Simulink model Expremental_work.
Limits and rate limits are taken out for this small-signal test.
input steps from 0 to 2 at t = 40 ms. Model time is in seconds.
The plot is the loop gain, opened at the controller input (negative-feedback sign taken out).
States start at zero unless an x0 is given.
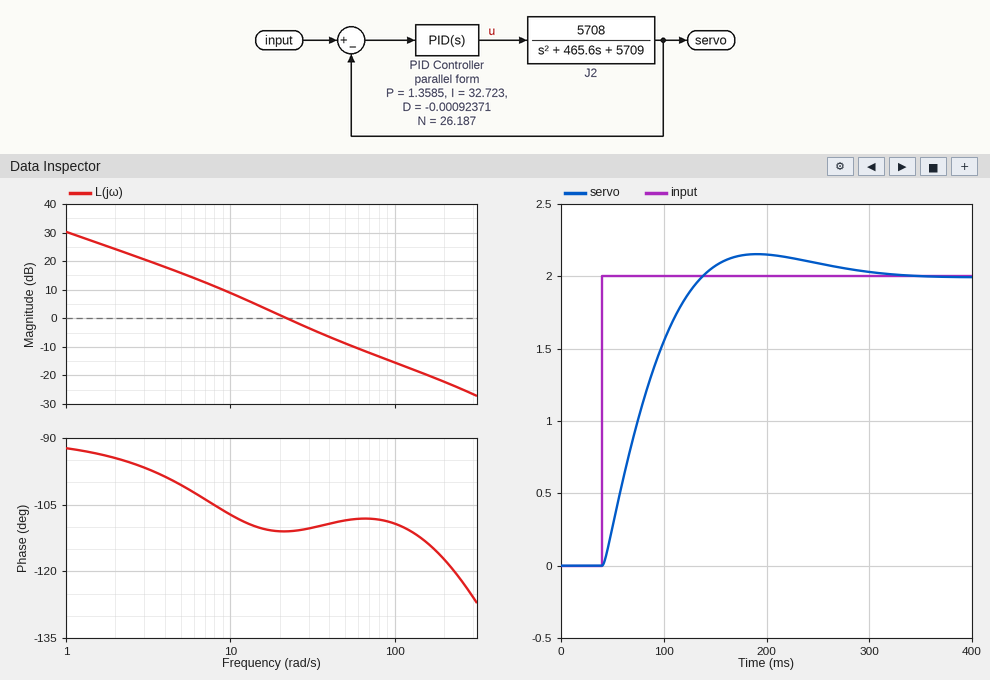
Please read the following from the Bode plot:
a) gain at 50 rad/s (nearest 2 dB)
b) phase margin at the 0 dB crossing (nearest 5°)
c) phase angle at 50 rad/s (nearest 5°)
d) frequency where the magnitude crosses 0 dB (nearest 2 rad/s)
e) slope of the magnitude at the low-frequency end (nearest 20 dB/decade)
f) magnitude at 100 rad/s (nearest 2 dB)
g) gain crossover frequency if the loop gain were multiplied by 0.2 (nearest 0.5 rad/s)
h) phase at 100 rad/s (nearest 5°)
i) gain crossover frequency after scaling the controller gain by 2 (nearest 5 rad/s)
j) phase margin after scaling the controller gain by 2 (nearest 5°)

-8 dB
70°
-110°
22 rad/s
-20 dB/decade
-16 dB
6.0 rad/s
-110°
40 rad/s
70°
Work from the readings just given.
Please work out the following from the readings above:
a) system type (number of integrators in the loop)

1
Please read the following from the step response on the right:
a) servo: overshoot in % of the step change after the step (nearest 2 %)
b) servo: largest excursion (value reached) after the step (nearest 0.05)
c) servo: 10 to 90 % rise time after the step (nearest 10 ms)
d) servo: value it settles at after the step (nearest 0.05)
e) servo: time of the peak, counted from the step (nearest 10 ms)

8 %
2.15
70 ms
2.00
150 ms
